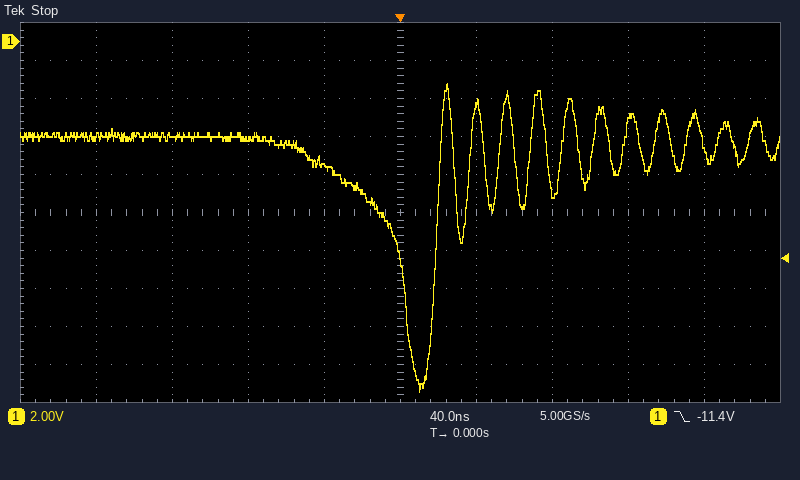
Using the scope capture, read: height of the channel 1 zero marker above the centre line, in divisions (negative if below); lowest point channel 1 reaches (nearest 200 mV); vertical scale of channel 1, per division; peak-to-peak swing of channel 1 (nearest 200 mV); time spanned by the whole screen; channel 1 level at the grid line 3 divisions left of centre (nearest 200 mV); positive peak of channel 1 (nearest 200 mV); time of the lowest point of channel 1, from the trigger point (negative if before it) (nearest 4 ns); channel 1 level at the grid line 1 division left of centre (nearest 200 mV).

+4.5 div
-18.4 V
2 V
16.2 V
400 ns
-5.0 V
-2.2 V
+12 ns
-6.6 V
